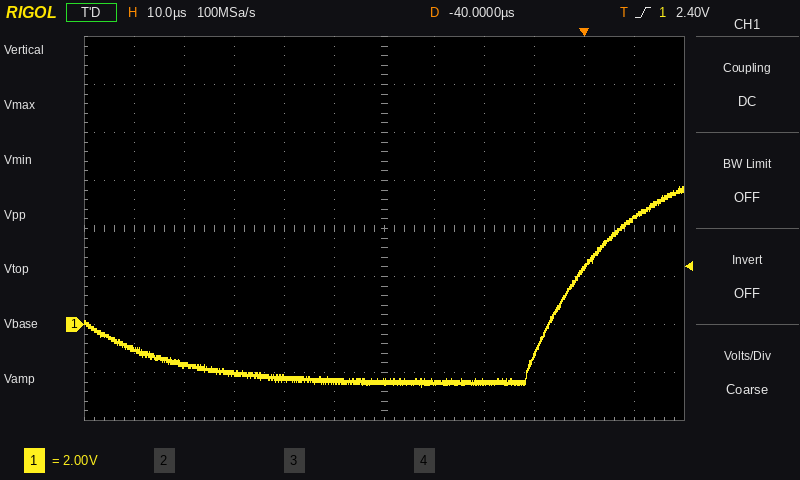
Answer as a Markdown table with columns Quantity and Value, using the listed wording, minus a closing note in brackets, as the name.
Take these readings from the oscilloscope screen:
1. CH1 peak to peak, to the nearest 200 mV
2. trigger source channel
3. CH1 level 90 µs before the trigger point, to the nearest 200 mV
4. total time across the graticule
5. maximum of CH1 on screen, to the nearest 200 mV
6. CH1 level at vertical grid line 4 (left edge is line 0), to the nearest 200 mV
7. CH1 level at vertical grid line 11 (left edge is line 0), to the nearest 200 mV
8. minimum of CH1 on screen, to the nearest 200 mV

| Quantity | Value |
|---|---|
| CH1 peak to peak, to the nearest 200 mV | 8.4 V |
| trigger source channel | CH1 |
| CH1 level 90 µs before the trigger point, to the nearest 200 mV | -1.0 V |
| total time across the graticule | 120 µs |
| maximum of CH1 on screen, to the nearest 200 mV | 5.8 V |
| CH1 level at vertical grid line 4 (left edge is line 0), to the nearest 200 mV | -2.2 V |
| CH1 level at vertical grid line 11 (left edge is line 0), to the nearest 200 mV | 4.4 V |
| minimum of CH1 on screen, to the nearest 200 mV | -2.6 V |
